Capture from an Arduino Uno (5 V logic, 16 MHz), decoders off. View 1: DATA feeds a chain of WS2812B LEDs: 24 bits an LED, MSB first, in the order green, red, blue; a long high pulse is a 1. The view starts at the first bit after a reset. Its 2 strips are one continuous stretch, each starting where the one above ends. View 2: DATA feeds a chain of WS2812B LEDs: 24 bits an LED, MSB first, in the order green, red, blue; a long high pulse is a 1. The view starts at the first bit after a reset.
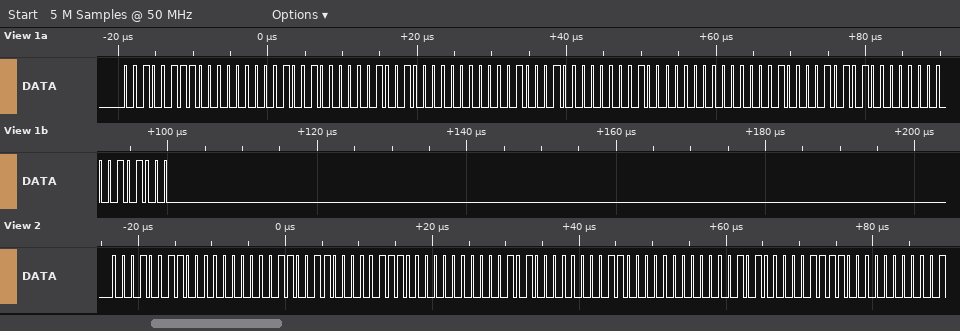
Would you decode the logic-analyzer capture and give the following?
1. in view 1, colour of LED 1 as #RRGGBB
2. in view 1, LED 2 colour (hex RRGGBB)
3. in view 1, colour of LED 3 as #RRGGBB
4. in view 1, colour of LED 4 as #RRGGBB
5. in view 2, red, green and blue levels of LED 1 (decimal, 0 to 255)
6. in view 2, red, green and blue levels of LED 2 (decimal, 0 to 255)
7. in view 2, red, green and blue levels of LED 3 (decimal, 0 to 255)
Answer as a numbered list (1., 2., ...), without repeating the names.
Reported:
1. #002748
2. #001222
3. #000102
4. #001528
5. 0, 19, 51
6. 0, 7, 20
7. 0, 3, 10
